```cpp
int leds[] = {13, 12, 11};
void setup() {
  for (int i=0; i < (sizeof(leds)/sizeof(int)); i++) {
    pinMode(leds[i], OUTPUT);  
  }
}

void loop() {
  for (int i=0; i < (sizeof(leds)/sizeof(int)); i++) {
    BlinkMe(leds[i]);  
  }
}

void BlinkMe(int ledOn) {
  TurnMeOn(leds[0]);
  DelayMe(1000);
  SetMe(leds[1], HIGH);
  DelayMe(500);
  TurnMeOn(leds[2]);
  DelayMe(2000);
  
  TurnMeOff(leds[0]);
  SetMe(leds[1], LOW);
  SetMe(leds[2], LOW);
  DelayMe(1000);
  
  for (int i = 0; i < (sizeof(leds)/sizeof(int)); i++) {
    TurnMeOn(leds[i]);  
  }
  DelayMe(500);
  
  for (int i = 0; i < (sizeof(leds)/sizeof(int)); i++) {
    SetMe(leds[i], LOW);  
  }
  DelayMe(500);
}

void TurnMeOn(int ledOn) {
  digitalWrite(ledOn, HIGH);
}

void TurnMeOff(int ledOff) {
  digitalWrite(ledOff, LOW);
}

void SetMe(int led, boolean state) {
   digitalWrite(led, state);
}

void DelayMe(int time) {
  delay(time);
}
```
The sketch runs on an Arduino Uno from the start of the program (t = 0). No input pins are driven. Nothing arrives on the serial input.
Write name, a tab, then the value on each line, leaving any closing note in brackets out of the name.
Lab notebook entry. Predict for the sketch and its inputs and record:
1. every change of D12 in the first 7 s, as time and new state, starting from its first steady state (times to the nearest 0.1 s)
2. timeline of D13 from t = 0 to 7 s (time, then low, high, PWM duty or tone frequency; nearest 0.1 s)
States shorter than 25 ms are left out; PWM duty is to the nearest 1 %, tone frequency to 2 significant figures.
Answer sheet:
every change of D12 in the first 7 s, as time and new state, starting from its first steady state	0 s low; 1 s high; 3.5 s low; 4.5 s high; 5 s low; 6.5 s high
timeline of D13 from t = 0 to 7 s	0 s high; 3.5 s low; 4.5 s high; 5 s low; 5.5 s high
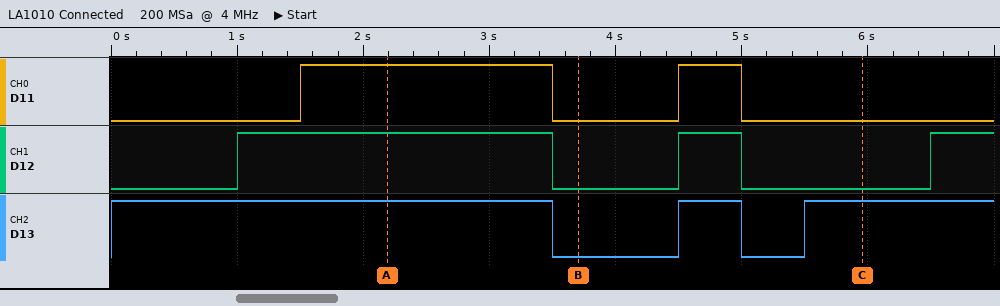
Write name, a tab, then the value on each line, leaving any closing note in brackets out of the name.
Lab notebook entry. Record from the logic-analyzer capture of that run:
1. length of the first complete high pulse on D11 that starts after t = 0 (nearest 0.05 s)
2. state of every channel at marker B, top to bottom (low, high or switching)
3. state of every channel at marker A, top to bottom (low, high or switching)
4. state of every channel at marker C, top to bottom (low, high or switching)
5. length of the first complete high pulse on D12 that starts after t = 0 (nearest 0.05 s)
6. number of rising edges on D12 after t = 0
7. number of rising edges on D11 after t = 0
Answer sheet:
length of the first complete high pulse on D11 that starts after t = 0	2.00 s
state of every channel at marker B, top to bottom	D11 low, D12 low, D13 low
state of every channel at marker A, top to bottom	D11 high, D12 high, D13 high
state of every channel at marker C, top to bottom	D11 low, D12 low, D13 high
length of the first complete high pulse on D12 that starts after t = 0	2.50 s
number of rising edges on D12 after t = 0	3
number of rising edges on D11 after t = 0	2
